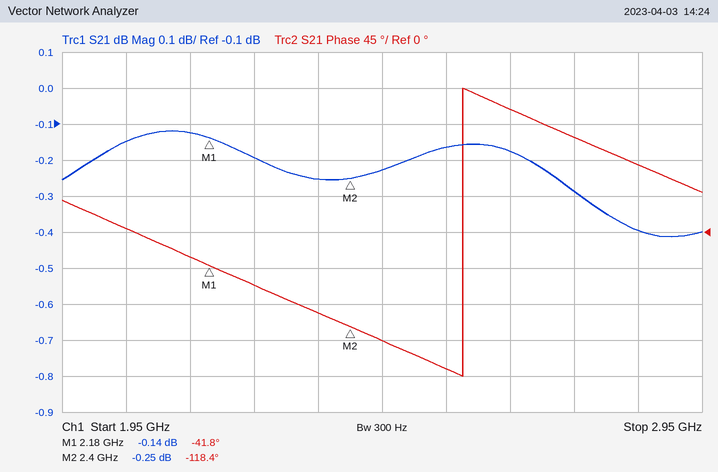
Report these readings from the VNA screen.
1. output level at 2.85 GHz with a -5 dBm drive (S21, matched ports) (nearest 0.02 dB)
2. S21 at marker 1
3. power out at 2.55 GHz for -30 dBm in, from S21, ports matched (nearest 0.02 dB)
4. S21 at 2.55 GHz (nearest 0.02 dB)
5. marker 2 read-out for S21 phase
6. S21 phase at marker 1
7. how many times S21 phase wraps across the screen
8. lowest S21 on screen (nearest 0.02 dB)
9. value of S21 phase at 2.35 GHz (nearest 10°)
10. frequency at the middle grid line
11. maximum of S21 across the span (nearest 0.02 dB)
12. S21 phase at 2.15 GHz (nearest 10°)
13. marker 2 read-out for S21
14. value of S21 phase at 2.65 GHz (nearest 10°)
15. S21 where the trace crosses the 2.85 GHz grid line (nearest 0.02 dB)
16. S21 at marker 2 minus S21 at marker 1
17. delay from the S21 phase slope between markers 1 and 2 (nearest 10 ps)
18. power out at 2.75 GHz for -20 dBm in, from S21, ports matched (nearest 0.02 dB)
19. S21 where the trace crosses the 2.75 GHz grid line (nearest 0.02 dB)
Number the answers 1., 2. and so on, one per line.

1. -5.40 dBm
2. -0.14 dB
3. -30.16 dBm
4. -0.16 dB
5. -118.4°
6. -41.8°
7. 1
8. -0.42 dB
9. -100°
10. 2.45 GHz
11. -0.12 dB
12. -30°
13. -0.25 dB
14. 150°
15. -0.40 dB
16. -0.11 dB
17. 970 ps
18. -20.28 dBm
19. -0.28 dB
